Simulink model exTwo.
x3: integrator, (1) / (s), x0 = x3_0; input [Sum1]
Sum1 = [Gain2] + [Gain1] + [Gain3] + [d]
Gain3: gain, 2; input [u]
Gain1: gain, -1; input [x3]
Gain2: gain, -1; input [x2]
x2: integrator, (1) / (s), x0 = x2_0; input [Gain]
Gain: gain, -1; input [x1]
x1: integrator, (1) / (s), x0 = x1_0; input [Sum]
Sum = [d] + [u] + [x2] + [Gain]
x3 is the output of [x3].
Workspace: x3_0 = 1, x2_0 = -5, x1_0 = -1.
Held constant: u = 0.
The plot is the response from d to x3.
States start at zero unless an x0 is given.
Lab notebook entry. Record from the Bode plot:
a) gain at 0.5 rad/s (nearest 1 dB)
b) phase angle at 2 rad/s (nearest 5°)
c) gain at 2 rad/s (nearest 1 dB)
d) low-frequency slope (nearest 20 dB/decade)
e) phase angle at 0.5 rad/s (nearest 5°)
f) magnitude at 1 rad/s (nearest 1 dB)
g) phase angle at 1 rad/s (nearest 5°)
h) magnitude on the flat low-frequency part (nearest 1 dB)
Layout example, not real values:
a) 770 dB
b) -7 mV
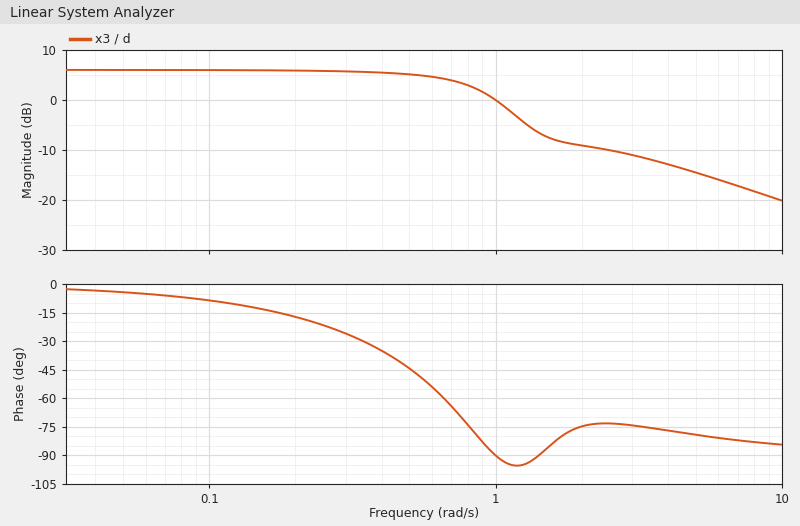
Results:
a) 5 dB
b) -75°
c) -9 dB
d) 0 dB/decade
e) -45°
f) 0 dB
g) -90°
h) 6 dB
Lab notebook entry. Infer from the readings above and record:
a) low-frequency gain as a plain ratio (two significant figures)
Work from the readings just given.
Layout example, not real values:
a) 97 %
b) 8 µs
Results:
a) 2.0
